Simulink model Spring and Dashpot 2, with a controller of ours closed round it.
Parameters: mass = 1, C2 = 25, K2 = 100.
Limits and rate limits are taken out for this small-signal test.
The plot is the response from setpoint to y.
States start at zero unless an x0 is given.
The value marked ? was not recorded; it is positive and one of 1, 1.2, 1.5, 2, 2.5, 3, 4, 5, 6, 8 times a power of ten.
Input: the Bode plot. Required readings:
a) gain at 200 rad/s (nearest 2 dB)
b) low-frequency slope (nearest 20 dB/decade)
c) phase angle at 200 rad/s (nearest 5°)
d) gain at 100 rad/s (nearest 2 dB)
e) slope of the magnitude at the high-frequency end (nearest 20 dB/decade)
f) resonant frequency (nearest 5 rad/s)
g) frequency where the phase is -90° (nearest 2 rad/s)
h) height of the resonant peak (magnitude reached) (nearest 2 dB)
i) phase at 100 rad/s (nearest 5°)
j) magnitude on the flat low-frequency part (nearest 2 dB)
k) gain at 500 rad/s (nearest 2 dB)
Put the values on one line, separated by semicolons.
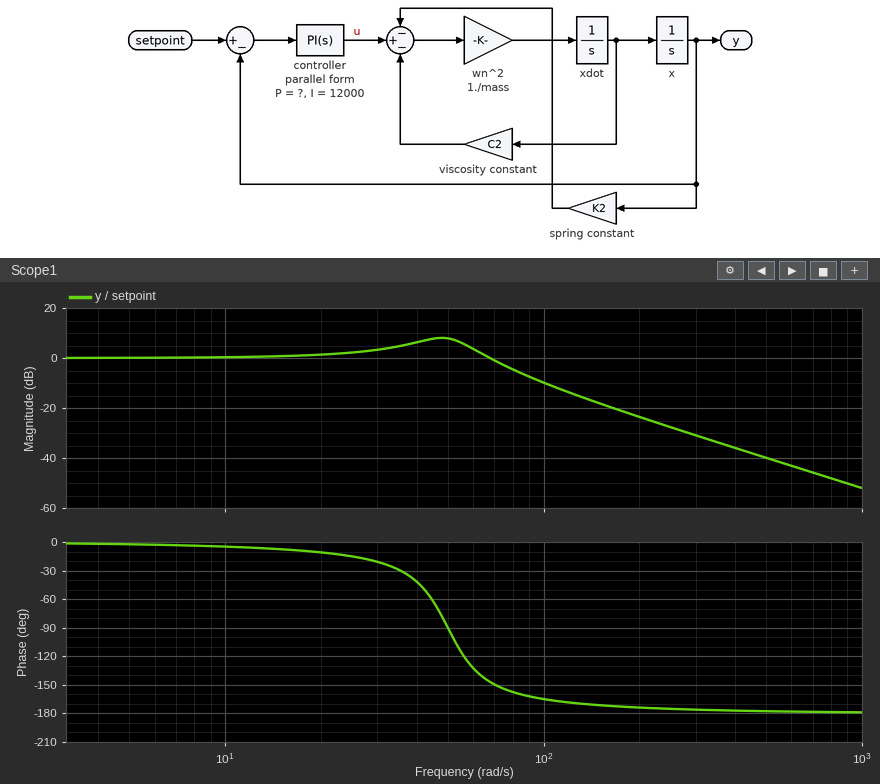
-24 dB; 0 dB/decade; -175°; -10 dB; -40 dB/decade; 50 rad/s; 50 rad/s; 8 dB; -165°; 0 dB; -40 dB
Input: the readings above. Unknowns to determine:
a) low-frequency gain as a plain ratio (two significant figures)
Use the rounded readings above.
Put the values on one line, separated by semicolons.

1.0
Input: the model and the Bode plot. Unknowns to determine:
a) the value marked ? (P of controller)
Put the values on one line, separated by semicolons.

2500
